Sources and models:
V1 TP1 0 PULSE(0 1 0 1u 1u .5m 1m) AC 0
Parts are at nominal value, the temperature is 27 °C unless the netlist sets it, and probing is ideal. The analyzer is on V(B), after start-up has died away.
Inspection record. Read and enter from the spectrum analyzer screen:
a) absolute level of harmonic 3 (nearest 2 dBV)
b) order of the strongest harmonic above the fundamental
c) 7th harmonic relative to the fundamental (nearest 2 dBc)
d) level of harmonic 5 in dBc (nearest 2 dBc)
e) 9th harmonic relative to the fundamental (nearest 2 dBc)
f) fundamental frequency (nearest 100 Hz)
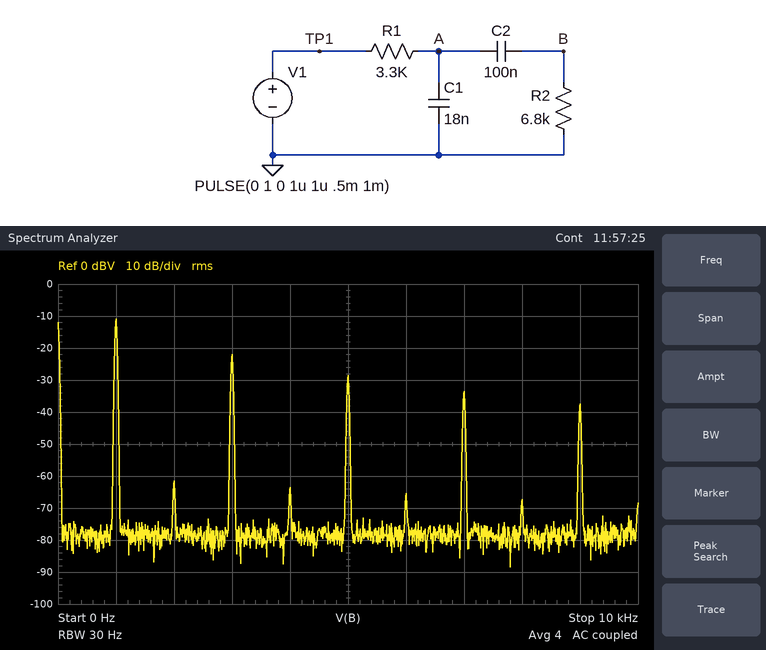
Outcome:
-22 dBV
3
-22 dBc
-18 dBc
-26 dBc
1.0 kHz
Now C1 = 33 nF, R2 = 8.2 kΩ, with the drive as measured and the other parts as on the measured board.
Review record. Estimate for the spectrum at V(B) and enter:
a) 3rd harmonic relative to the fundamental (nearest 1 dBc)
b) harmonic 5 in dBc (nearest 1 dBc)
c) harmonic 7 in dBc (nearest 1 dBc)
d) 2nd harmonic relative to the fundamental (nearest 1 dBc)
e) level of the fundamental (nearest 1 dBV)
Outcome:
-13 dBc
-21 dBc
-27 dBc
-52 dBc
-11 dBV
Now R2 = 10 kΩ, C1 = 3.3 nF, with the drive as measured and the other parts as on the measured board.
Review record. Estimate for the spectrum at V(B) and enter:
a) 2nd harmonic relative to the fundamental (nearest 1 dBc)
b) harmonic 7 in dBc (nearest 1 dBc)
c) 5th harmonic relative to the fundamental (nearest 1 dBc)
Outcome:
-50 dBc
-17 dBc
-14 dBc
